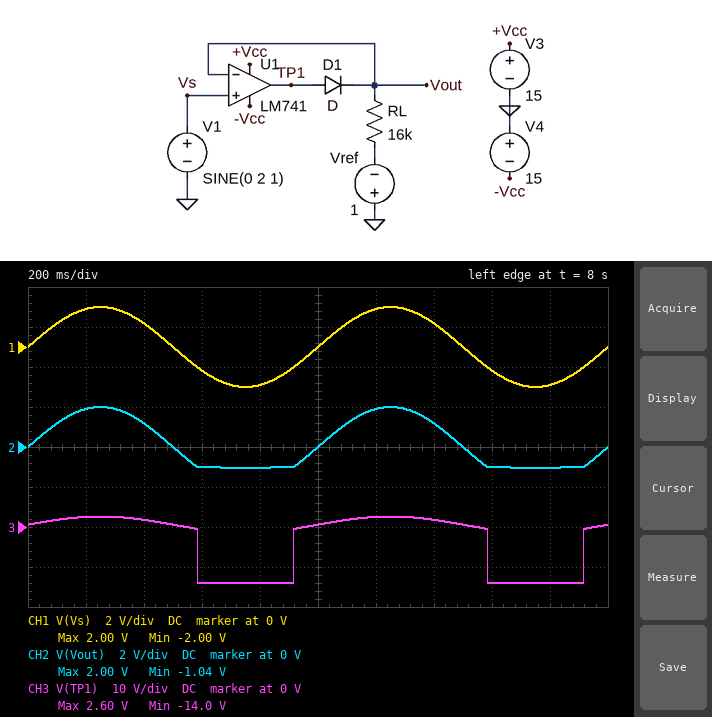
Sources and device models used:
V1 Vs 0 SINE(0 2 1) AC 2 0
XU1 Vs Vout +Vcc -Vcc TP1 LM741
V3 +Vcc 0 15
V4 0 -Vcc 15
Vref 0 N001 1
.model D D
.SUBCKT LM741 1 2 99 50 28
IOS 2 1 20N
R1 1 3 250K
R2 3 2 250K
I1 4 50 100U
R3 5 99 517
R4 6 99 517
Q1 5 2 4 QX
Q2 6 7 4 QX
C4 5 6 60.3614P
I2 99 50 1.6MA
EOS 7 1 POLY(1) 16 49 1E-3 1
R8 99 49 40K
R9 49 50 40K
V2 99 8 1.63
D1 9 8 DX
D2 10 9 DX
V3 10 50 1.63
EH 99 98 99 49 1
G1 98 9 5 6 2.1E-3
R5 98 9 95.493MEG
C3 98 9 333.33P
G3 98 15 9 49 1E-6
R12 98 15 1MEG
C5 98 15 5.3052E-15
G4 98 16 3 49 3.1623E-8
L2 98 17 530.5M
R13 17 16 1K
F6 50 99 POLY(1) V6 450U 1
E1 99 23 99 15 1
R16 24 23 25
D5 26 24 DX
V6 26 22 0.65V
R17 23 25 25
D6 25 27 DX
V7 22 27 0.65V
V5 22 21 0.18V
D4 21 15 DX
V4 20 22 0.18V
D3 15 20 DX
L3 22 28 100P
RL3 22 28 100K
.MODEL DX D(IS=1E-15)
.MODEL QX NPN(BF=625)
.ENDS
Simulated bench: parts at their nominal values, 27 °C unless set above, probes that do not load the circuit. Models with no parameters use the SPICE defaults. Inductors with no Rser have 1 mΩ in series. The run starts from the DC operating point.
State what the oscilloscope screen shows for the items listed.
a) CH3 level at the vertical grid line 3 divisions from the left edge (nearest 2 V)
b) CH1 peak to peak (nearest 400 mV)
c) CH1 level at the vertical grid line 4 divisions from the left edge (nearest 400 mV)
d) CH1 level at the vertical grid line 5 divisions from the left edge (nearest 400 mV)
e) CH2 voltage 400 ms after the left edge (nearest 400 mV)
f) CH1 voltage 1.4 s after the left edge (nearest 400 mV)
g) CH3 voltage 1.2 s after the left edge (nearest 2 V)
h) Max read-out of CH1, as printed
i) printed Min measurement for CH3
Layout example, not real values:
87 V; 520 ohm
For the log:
-14 V; 4.0 V; -2.0 V; 0 V; 1.2 V; 1.2 V; 2 V; 2.00 V; -14.0 V
